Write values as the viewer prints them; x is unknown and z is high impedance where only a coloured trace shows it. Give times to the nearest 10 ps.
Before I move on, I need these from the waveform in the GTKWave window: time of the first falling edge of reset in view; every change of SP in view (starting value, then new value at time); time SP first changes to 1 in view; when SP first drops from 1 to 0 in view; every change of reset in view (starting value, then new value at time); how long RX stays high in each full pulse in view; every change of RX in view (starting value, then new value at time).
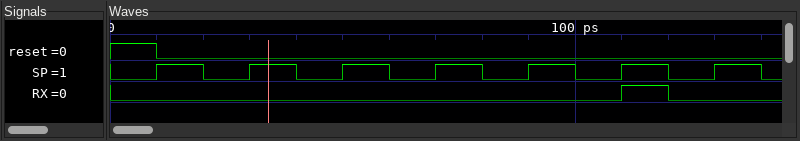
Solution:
10 ps
0, 1 at 10 ps, 0 at 20 ps, 1 at 30 ps, 0 at 40 ps, 1 at 50 ps, 0 at 60 ps, 1 at 70 ps, 0 at 80 ps, 1 at 90 ps, 0 at 100 ps, 1 at 110 ps, 0 at 120 ps, 1 at 130 ps, 0 at 140 ps
10 ps
20 ps
1, 0 at 10 ps
10 ps
0, 1 at 110 ps, 0 at 120 ps
